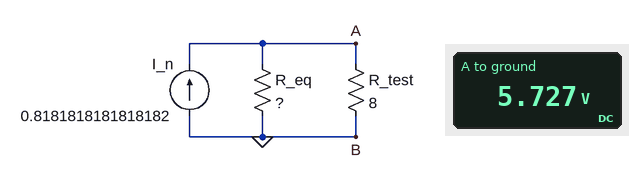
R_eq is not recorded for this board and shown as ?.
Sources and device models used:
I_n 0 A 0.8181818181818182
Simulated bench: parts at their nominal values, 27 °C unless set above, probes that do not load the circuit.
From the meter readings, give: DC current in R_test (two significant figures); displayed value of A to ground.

720 mA
5.727 V
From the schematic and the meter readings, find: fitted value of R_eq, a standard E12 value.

56 Ω
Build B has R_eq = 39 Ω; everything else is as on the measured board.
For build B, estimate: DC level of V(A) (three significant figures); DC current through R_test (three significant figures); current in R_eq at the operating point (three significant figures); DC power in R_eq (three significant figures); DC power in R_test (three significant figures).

5.43 V
679 mA
139 mA
756 mW
3.69 W
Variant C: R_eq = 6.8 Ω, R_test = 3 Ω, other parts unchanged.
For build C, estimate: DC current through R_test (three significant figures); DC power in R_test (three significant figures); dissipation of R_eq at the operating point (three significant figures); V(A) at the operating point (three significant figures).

568 mA
967 mW
427 mW
1.70 V
